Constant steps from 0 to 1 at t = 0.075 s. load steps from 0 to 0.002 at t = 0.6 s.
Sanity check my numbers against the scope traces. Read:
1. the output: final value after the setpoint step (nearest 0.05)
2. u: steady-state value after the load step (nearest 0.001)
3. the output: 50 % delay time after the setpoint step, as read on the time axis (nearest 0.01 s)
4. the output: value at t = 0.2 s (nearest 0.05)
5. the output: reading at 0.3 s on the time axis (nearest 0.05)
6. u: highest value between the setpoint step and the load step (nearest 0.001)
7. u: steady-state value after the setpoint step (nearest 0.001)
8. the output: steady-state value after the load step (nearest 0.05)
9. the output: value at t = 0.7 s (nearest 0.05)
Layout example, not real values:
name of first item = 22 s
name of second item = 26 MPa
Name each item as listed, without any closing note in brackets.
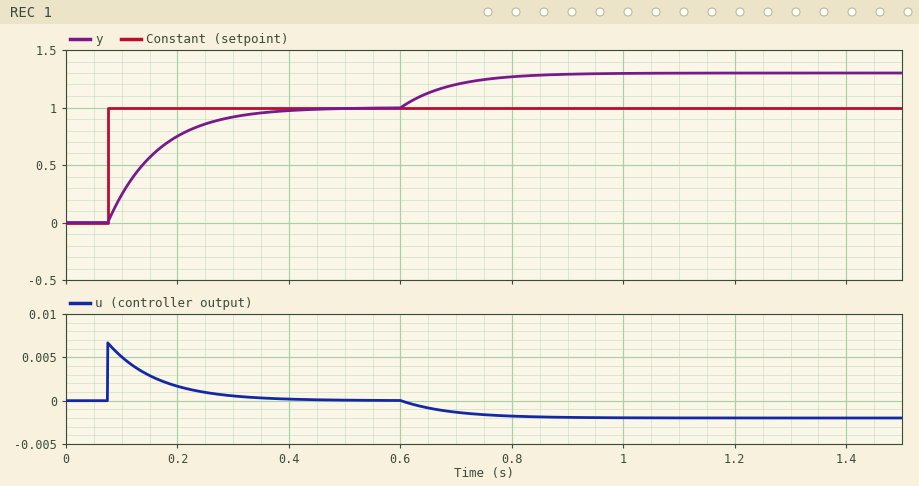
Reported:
the output: final value after the setpoint step = 1.00
u: steady-state value after the load step = -0.002
the output: 50 % delay time after the setpoint step, as read on the time axis = 0.14 s
the output: value at t = 0.2 s = 0.75
the output: reading at 0.3 s on the time axis = 0.90
u: highest value between the setpoint step and the load step = 0.007
u: steady-state value after the setpoint step = 0.000
the output: steady-state value after the load step = 1.30
the output: value at t = 0.7 s = 1.20
